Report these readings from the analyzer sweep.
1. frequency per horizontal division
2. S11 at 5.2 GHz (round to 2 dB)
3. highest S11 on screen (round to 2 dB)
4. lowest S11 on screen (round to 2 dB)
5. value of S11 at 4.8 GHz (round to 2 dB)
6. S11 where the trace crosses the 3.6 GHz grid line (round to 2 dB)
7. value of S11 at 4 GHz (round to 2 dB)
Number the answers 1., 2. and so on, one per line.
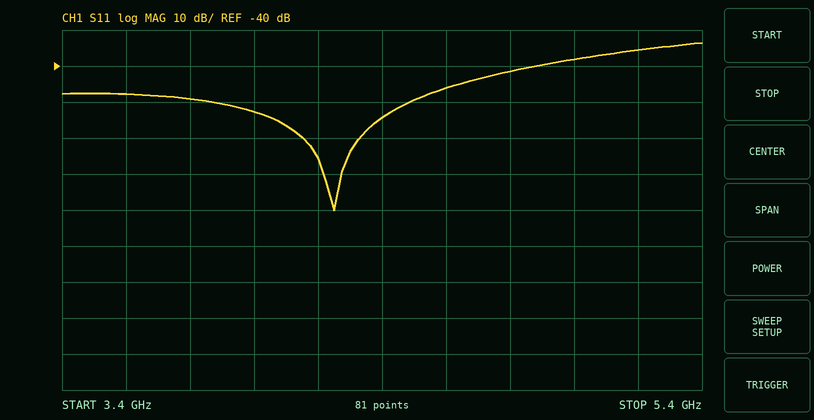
1. 200 MHz
2. -36 dB
3. -34 dB
4. -80 dB
5. -42 dB
6. -48 dB
7. -52 dB
